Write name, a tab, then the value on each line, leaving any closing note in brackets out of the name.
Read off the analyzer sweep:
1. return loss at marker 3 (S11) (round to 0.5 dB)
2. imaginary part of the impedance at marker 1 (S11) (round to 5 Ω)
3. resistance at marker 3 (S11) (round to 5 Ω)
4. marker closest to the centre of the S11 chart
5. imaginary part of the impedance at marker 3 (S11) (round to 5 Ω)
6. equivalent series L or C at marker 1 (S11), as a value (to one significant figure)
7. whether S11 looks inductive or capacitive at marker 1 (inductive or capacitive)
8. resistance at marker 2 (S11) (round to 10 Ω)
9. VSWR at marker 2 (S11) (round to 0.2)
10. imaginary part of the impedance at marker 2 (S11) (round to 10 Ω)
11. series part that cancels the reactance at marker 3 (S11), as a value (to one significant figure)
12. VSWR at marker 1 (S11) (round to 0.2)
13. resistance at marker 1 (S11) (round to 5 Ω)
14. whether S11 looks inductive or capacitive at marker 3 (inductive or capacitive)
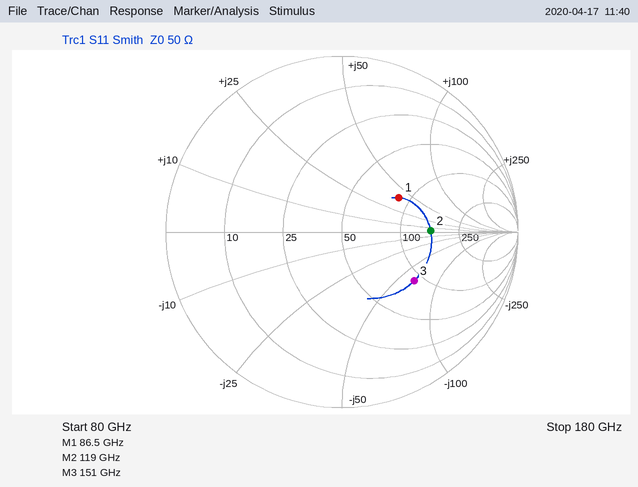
return loss at marker 3 (S11)	6.0 dB
imaginary part of the impedance at marker 1 (S11)	+40 Ω
resistance at marker 3 (S11)	90 Ω
marker closest to the centre of the S11 chart	marker 1
imaginary part of the impedance at marker 3 (S11)	-65 Ω
equivalent series L or C at marker 1 (S11), as a value	70 pH
whether S11 looks inductive or capacitive at marker 1	inductive
resistance at marker 2 (S11)	150 Ω
VSWR at marker 2 (S11)	3.0
imaginary part of the impedance at marker 2 (S11)	0 Ω
series part that cancels the reactance at marker 3 (S11), as a value	70 pH
VSWR at marker 1 (S11)	2.2
resistance at marker 1 (S11)	85 Ω
whether S11 looks inductive or capacitive at marker 3	capacitive
